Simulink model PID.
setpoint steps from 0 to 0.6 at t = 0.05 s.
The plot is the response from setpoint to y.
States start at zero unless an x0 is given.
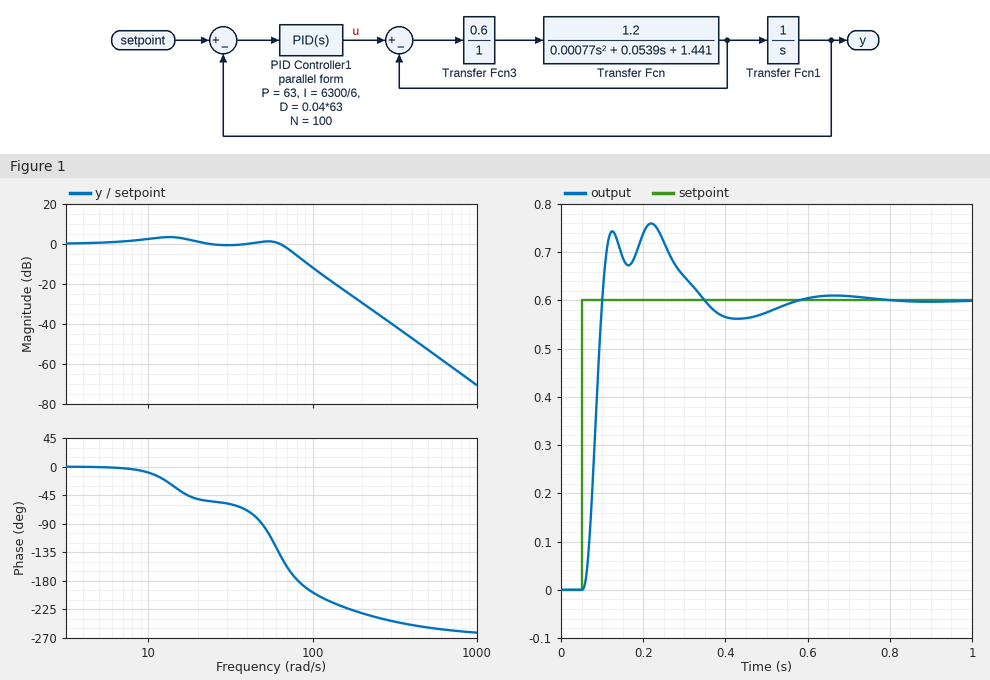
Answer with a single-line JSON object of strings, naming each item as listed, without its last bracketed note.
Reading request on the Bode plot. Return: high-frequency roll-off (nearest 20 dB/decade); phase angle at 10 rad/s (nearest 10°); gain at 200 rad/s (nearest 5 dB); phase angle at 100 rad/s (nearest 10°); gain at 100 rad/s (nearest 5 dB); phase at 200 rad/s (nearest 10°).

{"high-frequency roll-off": "-60 dB/decade", "phase angle at 10 rad/s": "-10°", "gain at 200 rad/s": "-30 dB", "phase angle at 100 rad/s": "-200°", "gain at 100 rad/s": "-10 dB", "phase at 200 rad/s": "-230°"}
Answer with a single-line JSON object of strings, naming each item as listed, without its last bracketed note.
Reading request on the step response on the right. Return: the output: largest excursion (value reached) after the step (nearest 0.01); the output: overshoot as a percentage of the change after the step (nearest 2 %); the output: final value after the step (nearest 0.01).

{"the output: largest excursion (value reached) after the step": "0.76", "the output: overshoot as a percentage of the change after the step": "26 %", "the output: final value after the step": "0.60"}
